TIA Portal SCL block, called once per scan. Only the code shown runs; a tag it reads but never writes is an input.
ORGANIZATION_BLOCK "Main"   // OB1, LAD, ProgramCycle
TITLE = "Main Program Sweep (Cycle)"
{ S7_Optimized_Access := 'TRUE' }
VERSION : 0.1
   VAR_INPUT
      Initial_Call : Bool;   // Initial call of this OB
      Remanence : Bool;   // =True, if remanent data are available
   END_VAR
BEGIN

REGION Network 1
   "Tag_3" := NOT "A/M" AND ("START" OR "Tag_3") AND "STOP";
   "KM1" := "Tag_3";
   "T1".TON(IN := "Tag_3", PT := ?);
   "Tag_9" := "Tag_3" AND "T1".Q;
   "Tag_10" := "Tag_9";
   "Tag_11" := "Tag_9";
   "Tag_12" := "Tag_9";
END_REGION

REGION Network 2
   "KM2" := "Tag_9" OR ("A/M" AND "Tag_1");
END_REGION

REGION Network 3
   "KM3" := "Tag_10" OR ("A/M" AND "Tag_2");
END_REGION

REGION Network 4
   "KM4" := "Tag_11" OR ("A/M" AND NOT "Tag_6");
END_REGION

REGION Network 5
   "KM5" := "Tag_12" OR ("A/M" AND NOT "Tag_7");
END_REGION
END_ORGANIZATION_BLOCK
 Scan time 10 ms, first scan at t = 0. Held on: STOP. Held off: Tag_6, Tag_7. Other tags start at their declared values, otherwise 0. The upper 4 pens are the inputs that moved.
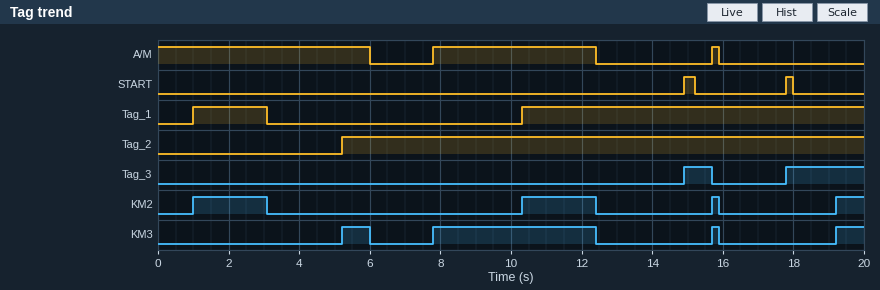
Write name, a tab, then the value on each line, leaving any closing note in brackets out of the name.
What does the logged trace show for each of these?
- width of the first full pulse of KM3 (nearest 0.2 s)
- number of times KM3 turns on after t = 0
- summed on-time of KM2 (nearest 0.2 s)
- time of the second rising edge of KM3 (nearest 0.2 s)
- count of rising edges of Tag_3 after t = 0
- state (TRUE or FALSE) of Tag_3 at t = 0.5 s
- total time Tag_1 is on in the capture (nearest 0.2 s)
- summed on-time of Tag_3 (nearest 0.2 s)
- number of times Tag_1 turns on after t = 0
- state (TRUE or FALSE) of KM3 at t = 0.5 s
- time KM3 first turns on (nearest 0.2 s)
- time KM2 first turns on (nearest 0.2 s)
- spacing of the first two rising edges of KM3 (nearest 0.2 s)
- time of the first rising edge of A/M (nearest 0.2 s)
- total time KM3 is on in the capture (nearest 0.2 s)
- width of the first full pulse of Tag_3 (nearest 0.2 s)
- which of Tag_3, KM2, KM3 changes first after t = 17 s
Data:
width of the first full pulse of KM3	0.8 s
number of times KM3 turns on after t = 0	4
summed on-time of KM2	5.2 s
time of the second rising edge of KM3	7.8 s
count of rising edges of Tag_3 after t = 0	2
state (TRUE or FALSE) of Tag_3 at t = 0.5 s	FALSE
total time Tag_1 is on in the capture	11.8 s
summed on-time of Tag_3	3.0 s
number of times Tag_1 turns on after t = 0	2
state (TRUE or FALSE) of KM3 at t = 0.5 s	FALSE
time KM3 first turns on	5.2 s
time KM2 first turns on	1.0 s
spacing of the first two rising edges of KM3	2.6 s
time of the first rising edge of A/M	7.8 s
total time KM3 is on in the capture	6.4 s
width of the first full pulse of Tag_3	0.8 s
which of Tag_3, KM2, KM3 changes first after t = 17 s	Tag_3
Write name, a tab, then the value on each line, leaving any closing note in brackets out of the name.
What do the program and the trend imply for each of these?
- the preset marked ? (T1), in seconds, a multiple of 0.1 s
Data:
the preset marked ? (T1), in seconds, a multiple of 0.1 s	1.4 s
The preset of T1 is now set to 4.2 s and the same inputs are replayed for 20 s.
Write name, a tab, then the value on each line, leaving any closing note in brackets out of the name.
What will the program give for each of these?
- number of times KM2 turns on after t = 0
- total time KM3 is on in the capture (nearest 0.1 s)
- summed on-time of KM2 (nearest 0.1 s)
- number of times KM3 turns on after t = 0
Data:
number of times KM2 turns on after t = 0	3
total time KM3 is on in the capture	5.6 s
summed on-time of KM2	4.4 s
number of times KM3 turns on after t = 0	3
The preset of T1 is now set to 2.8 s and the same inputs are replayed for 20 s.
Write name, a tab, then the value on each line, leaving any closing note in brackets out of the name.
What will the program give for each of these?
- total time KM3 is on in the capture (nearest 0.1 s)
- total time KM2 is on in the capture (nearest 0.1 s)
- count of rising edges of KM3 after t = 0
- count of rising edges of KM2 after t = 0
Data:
total time KM3 is on in the capture	5.6 s
total time KM2 is on in the capture	4.4 s
count of rising edges of KM3 after t = 0	3
count of rising edges of KM2 after t = 0	3
